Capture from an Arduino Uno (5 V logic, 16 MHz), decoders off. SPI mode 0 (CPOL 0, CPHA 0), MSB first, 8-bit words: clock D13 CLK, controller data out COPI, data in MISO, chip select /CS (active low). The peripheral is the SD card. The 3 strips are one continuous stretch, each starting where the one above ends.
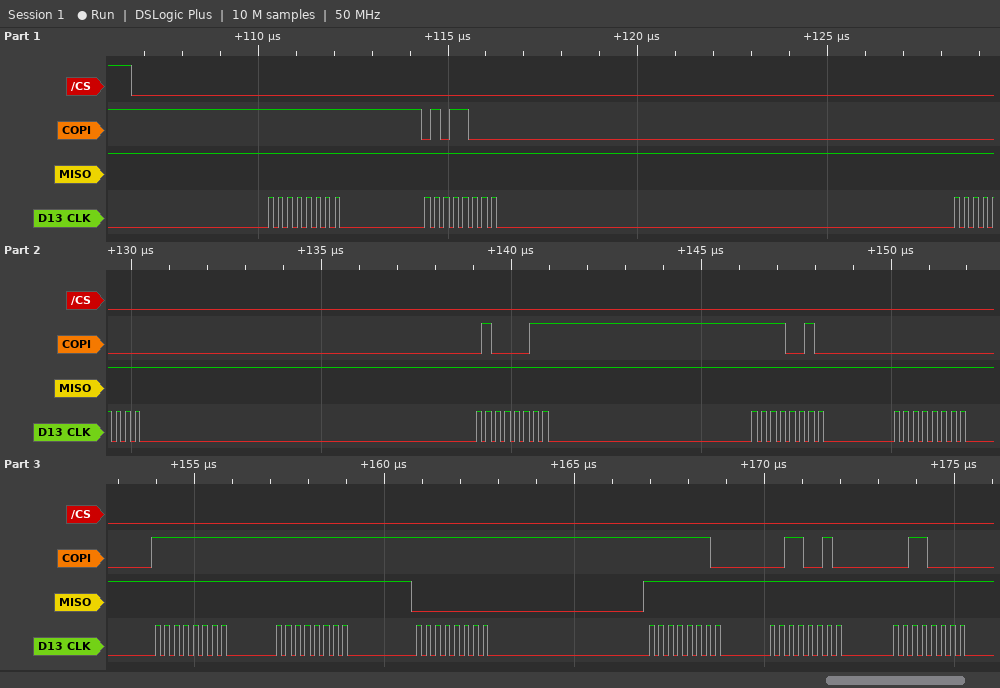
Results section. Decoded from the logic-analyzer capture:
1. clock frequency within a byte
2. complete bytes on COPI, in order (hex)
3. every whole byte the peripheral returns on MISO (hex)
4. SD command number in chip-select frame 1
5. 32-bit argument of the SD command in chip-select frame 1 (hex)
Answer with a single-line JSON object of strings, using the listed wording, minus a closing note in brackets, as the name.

{"clock frequency within a byte": "4 MHz", "complete bytes on COPI, in order": "FF 58 00 43 F2 00 FF FF FF FE 32 30", "every whole byte the peripheral returns on MISO": "FF FF FF FF FF FF FF FF 00 FF FF FF", "SD command number in chip-select frame 1": "CMD24", "32-bit argument of the SD command in chip-select frame 1": "0x0043F200"}
